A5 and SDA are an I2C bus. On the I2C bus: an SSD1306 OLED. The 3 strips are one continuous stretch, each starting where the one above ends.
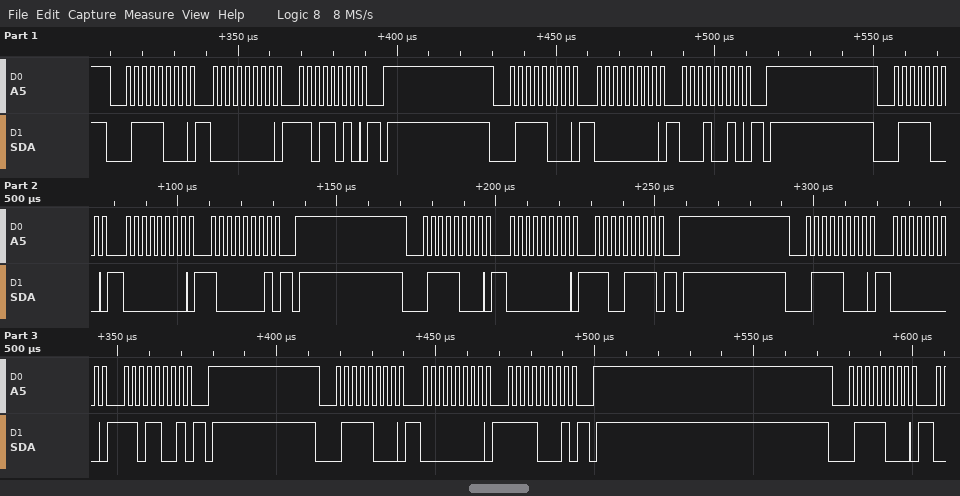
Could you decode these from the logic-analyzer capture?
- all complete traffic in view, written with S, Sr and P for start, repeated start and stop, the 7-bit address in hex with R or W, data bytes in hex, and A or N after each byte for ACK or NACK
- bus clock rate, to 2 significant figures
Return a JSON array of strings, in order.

["S 3CW A 00 A DA A P S 3CW A 00 A 12 A P S 3CW A 00 A 81 A P S 3CW A 00 A CF A P S 3CW A 00 A D9 A P S 3CW A 00 A F1 A P S 3CW A", "400 kHz"]
